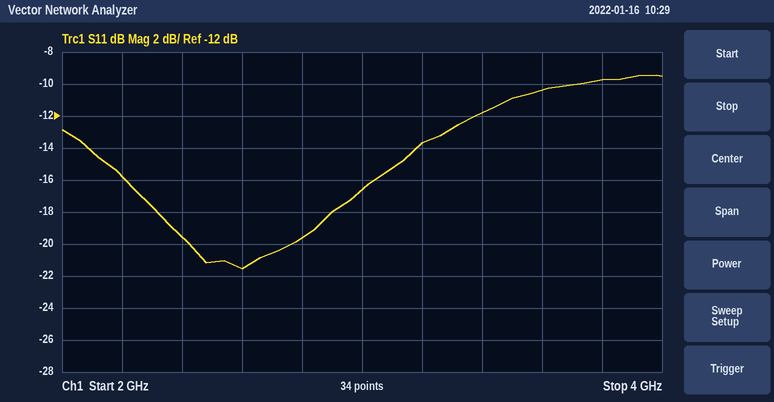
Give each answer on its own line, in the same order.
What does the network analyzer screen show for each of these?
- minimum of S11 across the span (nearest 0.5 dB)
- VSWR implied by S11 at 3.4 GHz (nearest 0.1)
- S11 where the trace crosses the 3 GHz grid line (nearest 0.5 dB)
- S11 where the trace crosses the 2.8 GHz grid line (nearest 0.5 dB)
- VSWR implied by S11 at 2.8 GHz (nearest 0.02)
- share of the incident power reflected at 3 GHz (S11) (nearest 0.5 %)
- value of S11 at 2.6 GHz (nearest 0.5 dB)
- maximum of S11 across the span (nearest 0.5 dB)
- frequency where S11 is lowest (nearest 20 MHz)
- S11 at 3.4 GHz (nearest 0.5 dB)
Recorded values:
-21.5 dB
1.7
-16.5 dB
-19.5 dB
1.24
2.0 %
-21.5 dB
-9.5 dB
2.60 GHz
-12.0 dB
